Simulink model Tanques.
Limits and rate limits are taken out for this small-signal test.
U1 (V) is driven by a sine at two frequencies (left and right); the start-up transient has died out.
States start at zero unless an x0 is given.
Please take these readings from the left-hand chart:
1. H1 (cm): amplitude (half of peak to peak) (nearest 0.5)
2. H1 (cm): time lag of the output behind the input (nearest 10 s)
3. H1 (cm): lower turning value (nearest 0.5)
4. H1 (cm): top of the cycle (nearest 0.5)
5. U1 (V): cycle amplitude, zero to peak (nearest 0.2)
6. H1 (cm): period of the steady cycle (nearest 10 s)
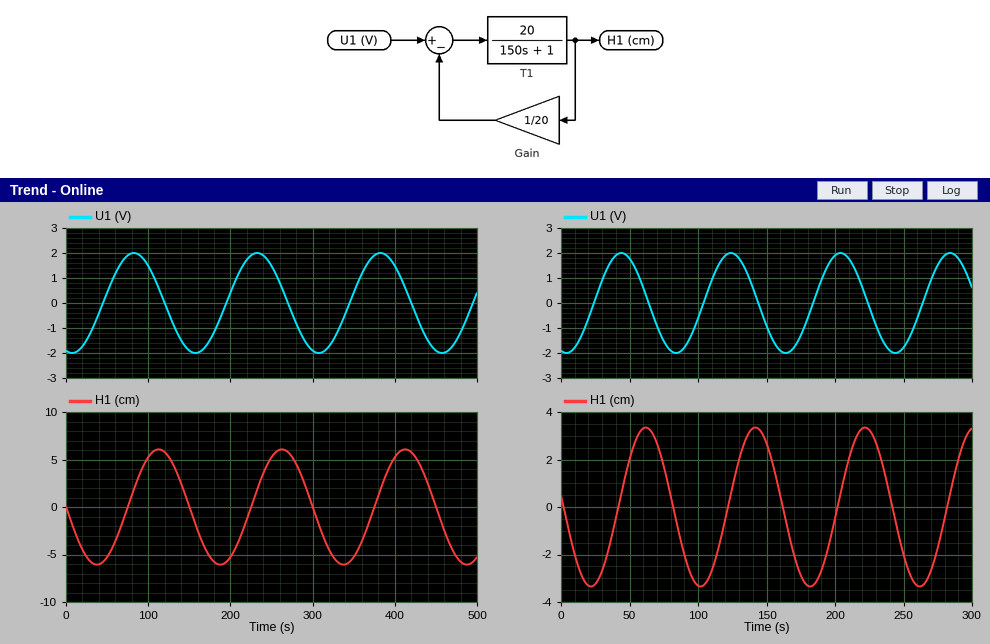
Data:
6.0
30 s
-6.0
6.0
2.0
150 s
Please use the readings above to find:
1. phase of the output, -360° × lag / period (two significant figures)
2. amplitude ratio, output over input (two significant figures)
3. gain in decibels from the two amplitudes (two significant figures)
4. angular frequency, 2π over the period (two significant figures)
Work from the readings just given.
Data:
-72°
3.0
9.5 dB
0.042 rad/s
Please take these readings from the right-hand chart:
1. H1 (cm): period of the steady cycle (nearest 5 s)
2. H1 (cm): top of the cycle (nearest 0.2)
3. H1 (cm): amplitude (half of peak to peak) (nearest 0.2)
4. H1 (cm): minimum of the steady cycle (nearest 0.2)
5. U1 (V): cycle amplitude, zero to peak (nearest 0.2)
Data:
80 s
3.4
3.4
-3.4
2.0
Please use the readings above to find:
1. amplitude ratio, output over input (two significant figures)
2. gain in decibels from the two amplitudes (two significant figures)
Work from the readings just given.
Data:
1.7
4.6 dB
